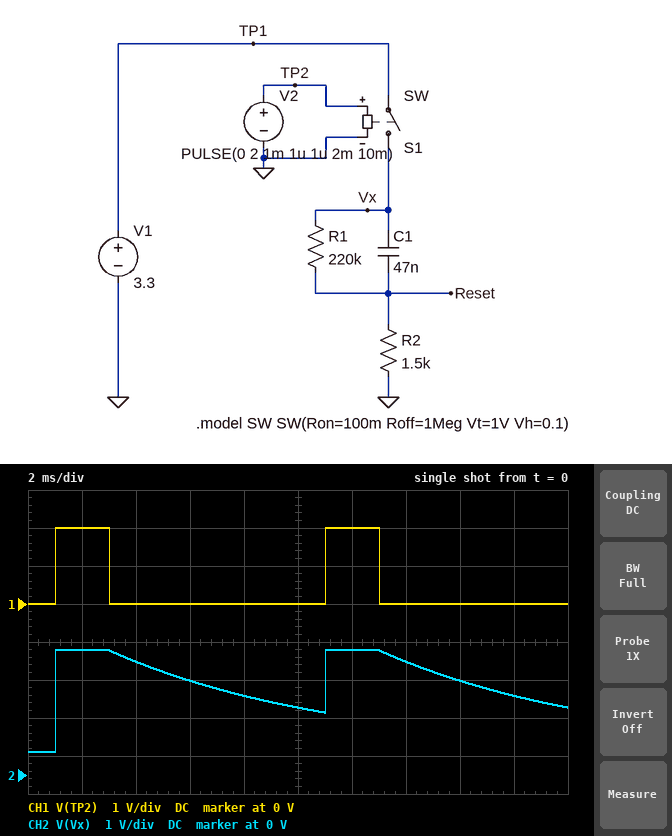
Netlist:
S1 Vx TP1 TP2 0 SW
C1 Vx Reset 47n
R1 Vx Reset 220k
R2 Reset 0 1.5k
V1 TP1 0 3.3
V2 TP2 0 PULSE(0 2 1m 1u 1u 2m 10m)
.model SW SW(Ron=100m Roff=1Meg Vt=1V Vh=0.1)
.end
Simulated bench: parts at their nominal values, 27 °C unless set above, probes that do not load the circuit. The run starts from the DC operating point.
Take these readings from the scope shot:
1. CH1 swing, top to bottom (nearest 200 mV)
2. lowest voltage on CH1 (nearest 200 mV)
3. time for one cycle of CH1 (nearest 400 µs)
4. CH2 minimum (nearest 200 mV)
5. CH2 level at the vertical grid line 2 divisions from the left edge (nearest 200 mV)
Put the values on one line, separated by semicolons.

2.0 V; 0 V; 10.0 ms; 600 mV; 3.0 V
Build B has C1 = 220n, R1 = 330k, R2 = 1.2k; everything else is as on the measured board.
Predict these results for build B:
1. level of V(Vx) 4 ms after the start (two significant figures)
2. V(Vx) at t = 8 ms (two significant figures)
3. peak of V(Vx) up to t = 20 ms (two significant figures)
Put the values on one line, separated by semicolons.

3.2 V; 3.1 V; 3.3 V
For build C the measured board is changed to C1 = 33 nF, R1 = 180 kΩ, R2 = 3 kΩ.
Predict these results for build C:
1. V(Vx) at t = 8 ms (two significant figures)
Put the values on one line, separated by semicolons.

1.5 V
